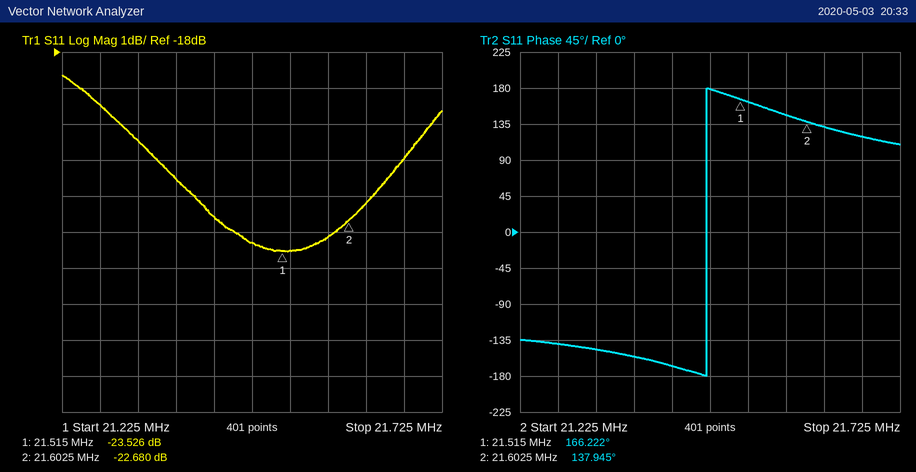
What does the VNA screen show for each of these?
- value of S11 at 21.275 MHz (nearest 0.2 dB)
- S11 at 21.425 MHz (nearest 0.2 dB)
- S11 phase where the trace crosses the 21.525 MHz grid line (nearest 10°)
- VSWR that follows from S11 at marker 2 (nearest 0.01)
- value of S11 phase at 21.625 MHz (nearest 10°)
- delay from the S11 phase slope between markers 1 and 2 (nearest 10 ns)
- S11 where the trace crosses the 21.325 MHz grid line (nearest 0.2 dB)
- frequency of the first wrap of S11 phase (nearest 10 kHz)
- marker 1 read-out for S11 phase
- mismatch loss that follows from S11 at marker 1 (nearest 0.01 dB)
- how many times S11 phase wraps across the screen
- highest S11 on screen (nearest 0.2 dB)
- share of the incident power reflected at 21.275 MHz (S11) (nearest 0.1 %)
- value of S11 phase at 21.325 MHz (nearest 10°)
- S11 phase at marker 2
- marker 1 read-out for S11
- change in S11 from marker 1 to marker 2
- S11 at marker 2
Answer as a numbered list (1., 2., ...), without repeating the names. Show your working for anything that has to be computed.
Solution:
1. -19.4 dB
2. -22.6 dB
3. 160°
4. (1 + 0.0735)/(1 − 0.0735) ≈ 1.16
5. 130°
6. −(137.945° − (166.222°))/(360° × 87.5 kHz) ≈ 898 ns, so 900 ns to the nearest 10 ns
7. -20.4 dB
8. 21.47 MHz
9. 166.222°
10. −10 log10(1 − 10^(-23.526/10)) ≈ 0.02 dB
11. 1
12. -18.6 dB
13. 10^(-19.4/10) ≈ 1.1 %
14. -150°
15. 137.945°
16. -23.526 dB
17. -22.68 − (-23.526) = 0.846 dB
18. -22.680 dB
